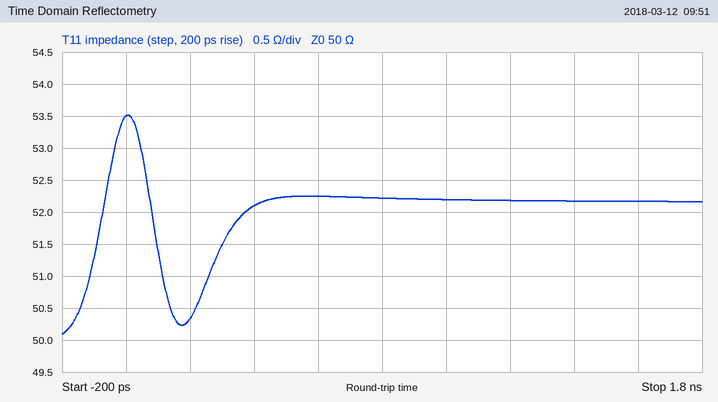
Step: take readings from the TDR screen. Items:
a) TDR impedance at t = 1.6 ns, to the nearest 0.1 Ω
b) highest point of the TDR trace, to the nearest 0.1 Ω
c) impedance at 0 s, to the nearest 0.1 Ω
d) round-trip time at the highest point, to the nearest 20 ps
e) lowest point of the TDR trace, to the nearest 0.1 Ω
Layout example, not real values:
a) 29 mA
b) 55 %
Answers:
a) 52.2 Ω
b) 53.5 Ω
c) 53.5 Ω
d) 0 ps
e) 50.1 Ω
